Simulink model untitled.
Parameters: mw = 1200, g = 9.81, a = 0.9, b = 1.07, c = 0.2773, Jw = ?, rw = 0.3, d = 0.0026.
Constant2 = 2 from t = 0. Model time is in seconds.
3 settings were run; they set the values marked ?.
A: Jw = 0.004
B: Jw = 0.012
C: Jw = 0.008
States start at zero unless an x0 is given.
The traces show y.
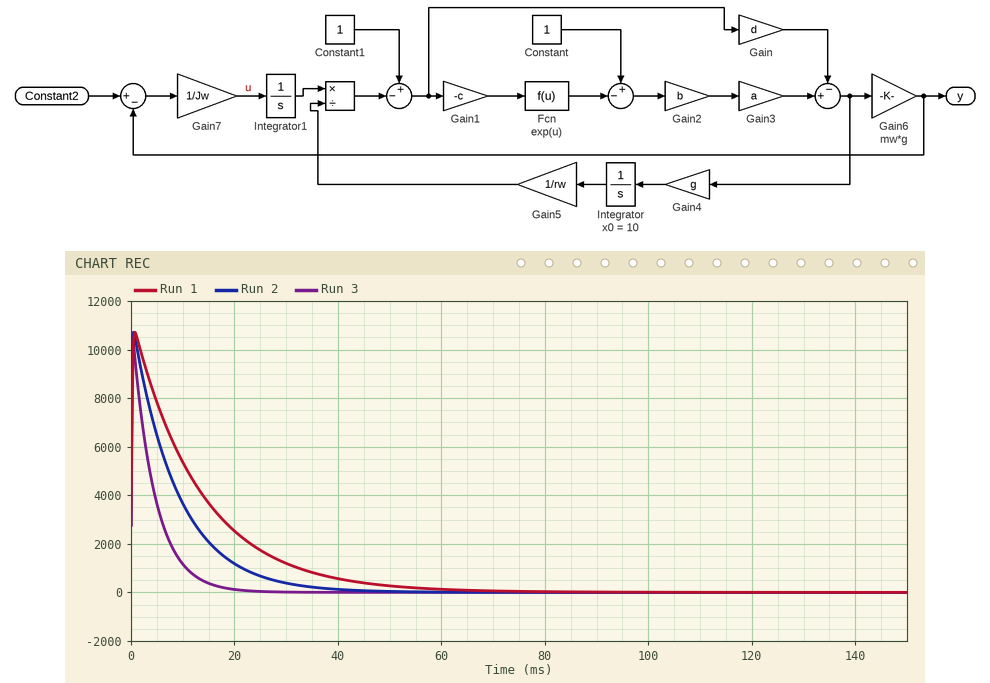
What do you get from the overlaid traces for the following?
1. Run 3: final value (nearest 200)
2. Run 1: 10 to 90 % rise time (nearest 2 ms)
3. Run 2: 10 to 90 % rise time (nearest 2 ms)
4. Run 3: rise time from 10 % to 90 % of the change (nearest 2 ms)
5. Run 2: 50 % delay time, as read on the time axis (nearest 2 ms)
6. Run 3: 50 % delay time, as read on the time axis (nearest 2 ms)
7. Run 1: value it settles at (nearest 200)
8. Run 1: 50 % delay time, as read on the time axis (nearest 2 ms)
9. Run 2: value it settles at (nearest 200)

0
30 ms
20 ms
10 ms
18 ms
10 ms
0
28 ms
0
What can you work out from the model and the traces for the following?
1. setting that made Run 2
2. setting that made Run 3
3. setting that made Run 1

C
A
B
